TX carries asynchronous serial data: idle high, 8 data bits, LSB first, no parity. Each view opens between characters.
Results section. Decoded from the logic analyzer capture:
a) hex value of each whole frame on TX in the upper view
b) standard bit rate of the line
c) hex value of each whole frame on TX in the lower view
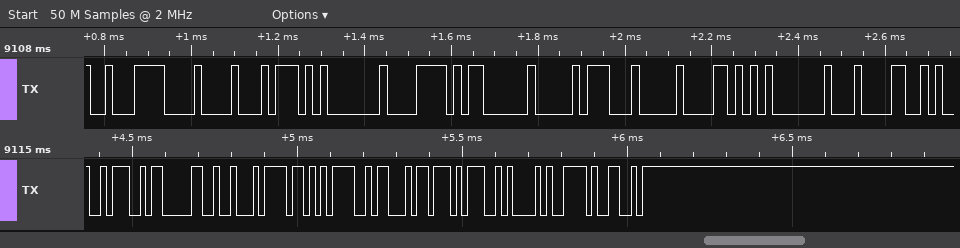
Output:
E2, 08, 74, 01, 78, 03, D0, 04, 58, 01, 84
57600 baud
3A, 83, 12, 6F, 3D, A3, D7, 0A, 79, A6
